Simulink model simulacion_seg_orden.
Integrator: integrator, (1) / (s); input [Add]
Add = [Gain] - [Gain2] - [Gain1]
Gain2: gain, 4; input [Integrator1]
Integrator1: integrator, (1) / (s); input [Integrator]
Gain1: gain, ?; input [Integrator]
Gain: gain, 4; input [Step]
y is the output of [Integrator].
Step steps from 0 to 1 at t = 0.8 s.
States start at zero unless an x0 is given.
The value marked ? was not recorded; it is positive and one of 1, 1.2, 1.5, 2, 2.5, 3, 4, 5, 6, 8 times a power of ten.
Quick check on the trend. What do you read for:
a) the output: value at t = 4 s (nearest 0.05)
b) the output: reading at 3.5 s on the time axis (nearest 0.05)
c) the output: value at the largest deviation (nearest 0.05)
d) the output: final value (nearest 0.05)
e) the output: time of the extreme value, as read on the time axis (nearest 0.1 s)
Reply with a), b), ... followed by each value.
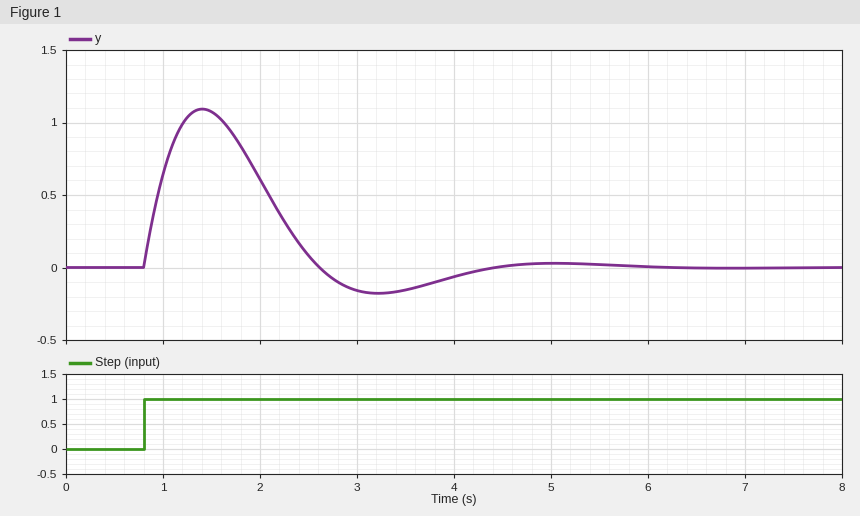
a) -0.05
b) -0.15
c) 1.10
d) 0.00
e) 1.4 s
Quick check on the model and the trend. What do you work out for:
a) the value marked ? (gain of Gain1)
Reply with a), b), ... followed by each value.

a) 2
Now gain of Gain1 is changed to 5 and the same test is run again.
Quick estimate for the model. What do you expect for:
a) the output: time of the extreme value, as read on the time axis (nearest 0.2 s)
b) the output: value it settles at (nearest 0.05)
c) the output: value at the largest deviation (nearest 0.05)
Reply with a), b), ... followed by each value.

a) 1.2 s
b) 0.00
c) 0.65
